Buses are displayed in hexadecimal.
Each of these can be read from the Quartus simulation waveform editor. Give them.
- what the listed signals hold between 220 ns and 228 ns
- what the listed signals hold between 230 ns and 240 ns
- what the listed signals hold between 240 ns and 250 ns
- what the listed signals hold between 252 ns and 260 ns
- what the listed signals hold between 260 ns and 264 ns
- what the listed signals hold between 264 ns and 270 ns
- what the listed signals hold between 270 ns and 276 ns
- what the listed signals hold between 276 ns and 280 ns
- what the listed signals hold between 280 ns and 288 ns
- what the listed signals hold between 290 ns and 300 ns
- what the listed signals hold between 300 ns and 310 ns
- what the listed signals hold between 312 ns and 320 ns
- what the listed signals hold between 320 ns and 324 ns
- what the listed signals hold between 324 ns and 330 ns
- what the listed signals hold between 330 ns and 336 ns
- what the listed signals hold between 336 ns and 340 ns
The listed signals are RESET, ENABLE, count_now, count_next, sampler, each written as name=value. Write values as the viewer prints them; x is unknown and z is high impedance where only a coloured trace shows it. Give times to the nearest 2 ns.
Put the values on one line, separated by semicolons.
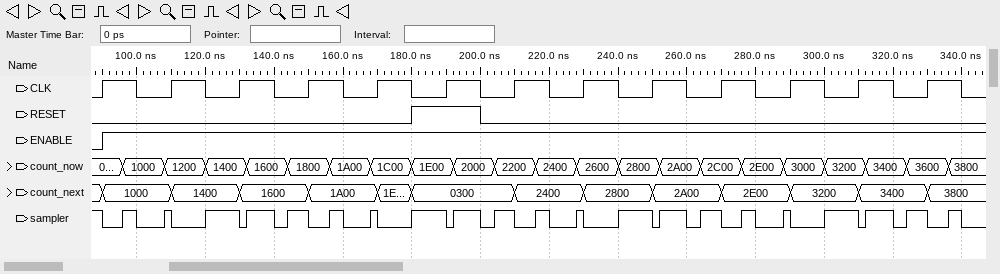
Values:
RESET=0, ENABLE=1, count_now=2400, count_next=2400, sampler=0; RESET=0, ENABLE=1, count_now=2600, count_next=2800, sampler=0; RESET=0, ENABLE=1, count_now=2800, count_next=2800, sampler=1; RESET=0, ENABLE=1, count_now=2A00, count_next=2A00, sampler=1; RESET=0, ENABLE=1, count_now=2A00, count_next=2A00, sampler=0; RESET=0, ENABLE=1, count_now=2C00, count_next=2A00, sampler=1; RESET=0, ENABLE=1, count_now=2C00, count_next=2E00, sampler=0; RESET=0, ENABLE=1, count_now=2E00, count_next=2E00, sampler=1; RESET=0, ENABLE=1, count_now=2E00, count_next=2E00, sampler=0; RESET=0, ENABLE=1, count_now=3000, count_next=3200, sampler=0; RESET=0, ENABLE=1, count_now=3200, count_next=3200, sampler=1; RESET=0, ENABLE=1, count_now=3400, count_next=3400, sampler=1; RESET=0, ENABLE=1, count_now=3400, count_next=3400, sampler=0; RESET=0, ENABLE=1, count_now=3600, count_next=3400, sampler=1; RESET=0, ENABLE=1, count_now=3600, count_next=3800, sampler=0; RESET=0, ENABLE=1, count_now=3800, count_next=3800, sampler=1
